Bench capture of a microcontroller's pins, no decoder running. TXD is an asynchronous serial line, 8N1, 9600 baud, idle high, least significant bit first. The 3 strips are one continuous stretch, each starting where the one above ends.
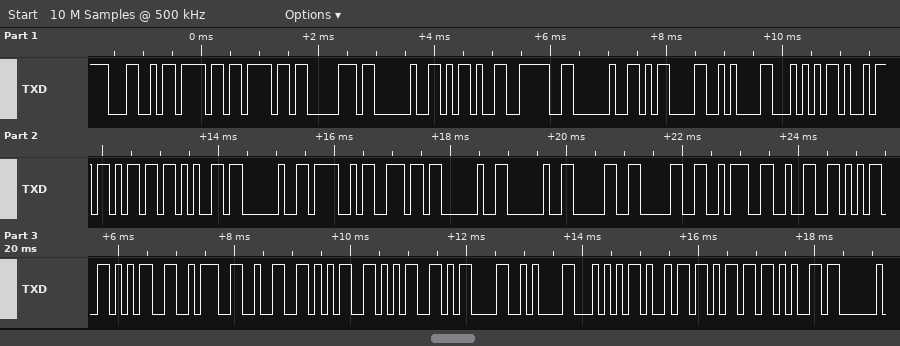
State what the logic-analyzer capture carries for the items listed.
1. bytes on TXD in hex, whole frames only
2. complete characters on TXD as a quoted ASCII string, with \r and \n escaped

4C 6F 6F 70 20 2D 3E 20 0D 0A 54 69 6D 65 20 4F 6E 20 20 30 30 3A 32 35 35 3A 32 35 35 0D 0A 54 69 6D 65
"Loop -> \r\nTime On  00:255:255\r\nTime"
